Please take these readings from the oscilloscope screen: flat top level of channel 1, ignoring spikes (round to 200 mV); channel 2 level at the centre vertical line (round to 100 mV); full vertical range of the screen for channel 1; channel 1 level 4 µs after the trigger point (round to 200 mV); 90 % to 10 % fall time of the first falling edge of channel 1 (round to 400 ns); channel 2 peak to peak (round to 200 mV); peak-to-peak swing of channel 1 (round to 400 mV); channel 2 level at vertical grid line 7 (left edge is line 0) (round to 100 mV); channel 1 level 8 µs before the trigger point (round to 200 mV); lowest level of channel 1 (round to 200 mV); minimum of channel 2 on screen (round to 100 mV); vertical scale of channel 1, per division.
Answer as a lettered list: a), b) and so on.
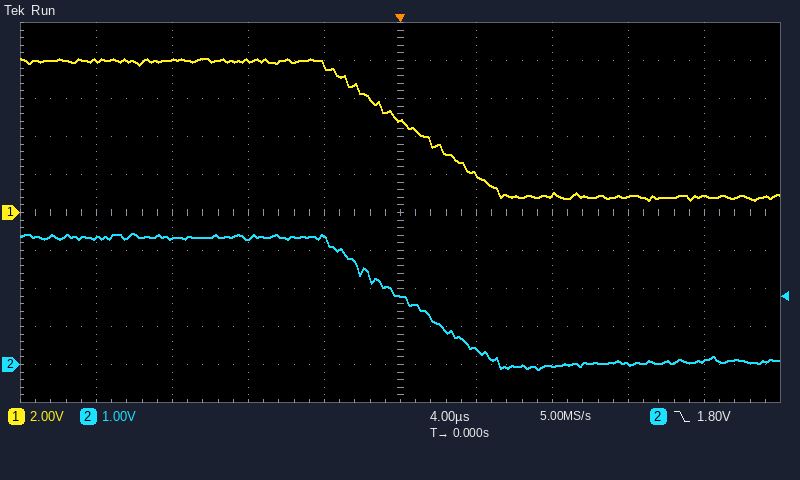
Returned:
a) 8.0 V
b) 1.8 V
c) 20 V
d) 2.0 V
e) 8.0 µs
f) 3.6 V
g) 7.6 V
h) 0.0 V
i) 8.0 V
j) 600 mV
k) -100 mV
l) 2 V
